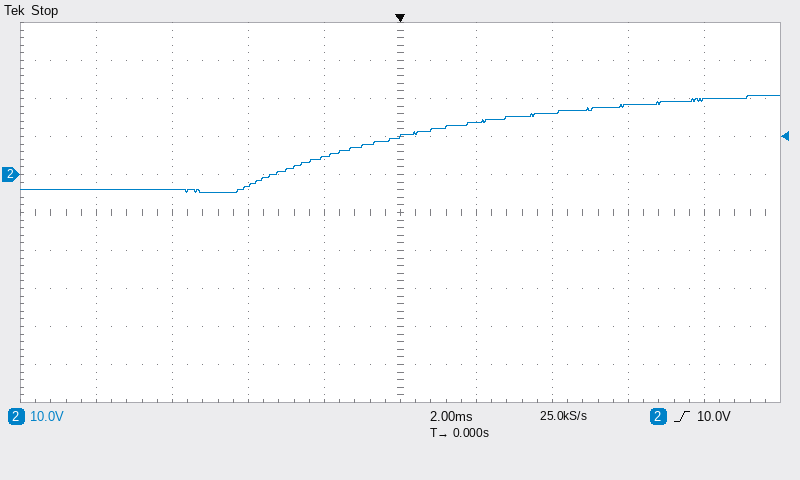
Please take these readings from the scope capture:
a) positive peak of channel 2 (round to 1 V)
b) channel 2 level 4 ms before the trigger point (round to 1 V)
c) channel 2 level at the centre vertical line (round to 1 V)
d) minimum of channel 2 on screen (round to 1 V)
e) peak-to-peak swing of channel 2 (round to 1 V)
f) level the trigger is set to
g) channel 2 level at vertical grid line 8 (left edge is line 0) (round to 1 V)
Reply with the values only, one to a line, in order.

21 V
-3 V
10 V
-5 V
26 V
10.0 V
18 V
